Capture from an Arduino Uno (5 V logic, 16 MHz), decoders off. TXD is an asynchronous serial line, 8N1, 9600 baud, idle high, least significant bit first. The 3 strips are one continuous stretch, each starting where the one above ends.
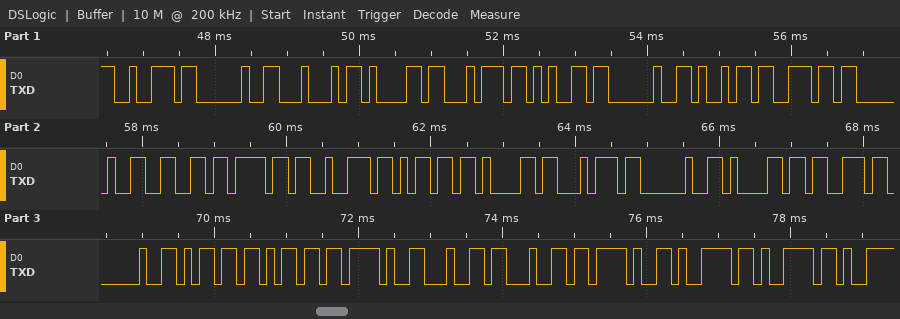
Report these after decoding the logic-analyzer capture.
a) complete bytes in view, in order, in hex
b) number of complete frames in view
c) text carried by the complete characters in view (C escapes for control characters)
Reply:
72 20 44 61 74 65 20 69 6E 20 66 6F 72 6D 61 74 20 61 73 20 6D 6D 2F 64 64 2F 79 79
28
"r Date in format as mm/dd/yy"
